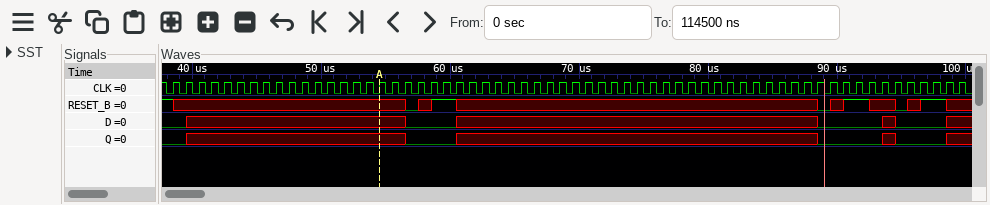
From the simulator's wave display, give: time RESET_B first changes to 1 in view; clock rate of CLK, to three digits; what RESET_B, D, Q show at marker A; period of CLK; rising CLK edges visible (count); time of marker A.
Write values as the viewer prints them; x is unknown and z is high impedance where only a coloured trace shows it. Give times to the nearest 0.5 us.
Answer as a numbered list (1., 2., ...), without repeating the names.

1. 58.5 us
2. 1.00 MHz
3. RESET_B=x, D=x, Q=x
4. 1 us
5. 62
6. 54.5 us
